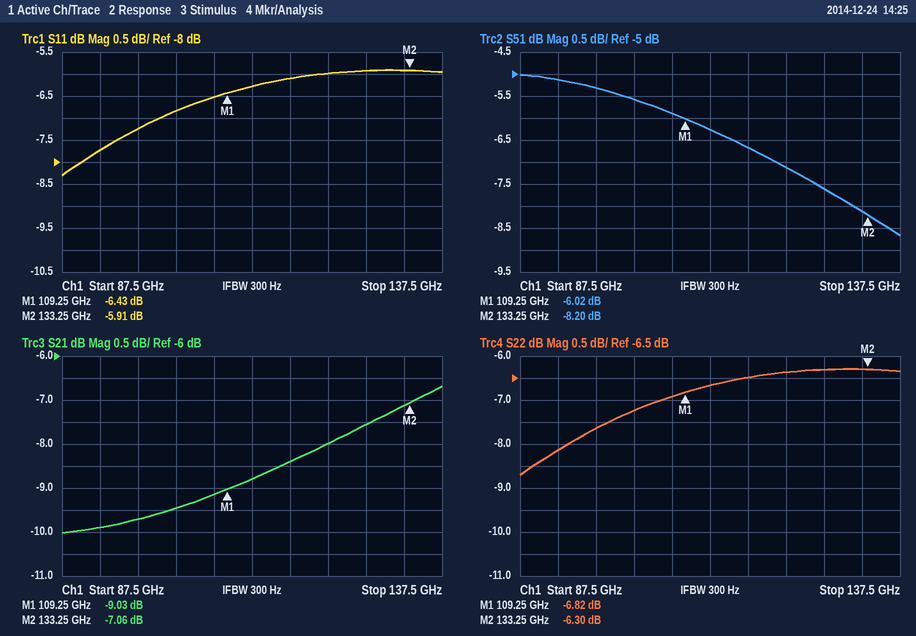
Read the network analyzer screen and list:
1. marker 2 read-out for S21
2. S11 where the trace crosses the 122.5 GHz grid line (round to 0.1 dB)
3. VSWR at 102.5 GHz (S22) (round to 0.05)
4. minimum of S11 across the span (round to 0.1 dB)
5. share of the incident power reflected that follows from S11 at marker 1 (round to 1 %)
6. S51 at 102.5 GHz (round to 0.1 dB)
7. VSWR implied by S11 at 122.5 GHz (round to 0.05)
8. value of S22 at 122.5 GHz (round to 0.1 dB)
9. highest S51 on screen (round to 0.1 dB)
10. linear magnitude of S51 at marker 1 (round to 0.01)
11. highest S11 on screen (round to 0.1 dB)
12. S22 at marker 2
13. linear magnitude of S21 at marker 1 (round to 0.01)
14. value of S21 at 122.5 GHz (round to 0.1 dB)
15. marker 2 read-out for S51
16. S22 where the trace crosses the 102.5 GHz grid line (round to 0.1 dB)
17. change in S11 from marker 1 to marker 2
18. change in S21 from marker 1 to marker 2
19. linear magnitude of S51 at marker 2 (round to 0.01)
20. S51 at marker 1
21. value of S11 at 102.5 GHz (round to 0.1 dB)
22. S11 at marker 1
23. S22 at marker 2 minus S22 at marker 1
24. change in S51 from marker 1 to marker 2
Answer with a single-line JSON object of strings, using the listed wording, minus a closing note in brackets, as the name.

{"marker 2 read-out for S21": "-7.06 dB", "S11 where the trace crosses the 122.5 GHz grid line": "-6.0 dB", "VSWR at 102.5 GHz (S22)": "2.55", "minimum of S11 across the span": "-8.3 dB", "share of the incident power reflected that follows from S11 at marker 1": "23 %", "S51 at 102.5 GHz": "-5.6 dB", "VSWR implied by S11 at 122.5 GHz": "3.00", "value of S22 at 122.5 GHz": "-6.4 dB", "highest S51 on screen": "-5.0 dB", "linear magnitude of S51 at marker 1": "0.50", "highest S11 on screen": "-5.9 dB", "S22 at marker 2": "-6.30 dB", "linear magnitude of S21 at marker 1": "0.35", "value of S21 at 122.5 GHz": "-8.0 dB", "marker 2 read-out for S51": "-8.20 dB", "S22 where the trace crosses the 102.5 GHz grid line": "-7.2 dB", "change in S11 from marker 1 to marker 2": "0.52 dB", "change in S21 from marker 1 to marker 2": "1.97 dB", "linear magnitude of S51 at marker 2": "0.39", "S51 at marker 1": "-6.02 dB", "value of S11 at 102.5 GHz": "-6.8 dB", "S11 at marker 1": "-6.43 dB", "S22 at marker 2 minus S22 at marker 1": "0.52 dB", "change in S51 from marker 1 to marker 2": "-2.18 dB"}
